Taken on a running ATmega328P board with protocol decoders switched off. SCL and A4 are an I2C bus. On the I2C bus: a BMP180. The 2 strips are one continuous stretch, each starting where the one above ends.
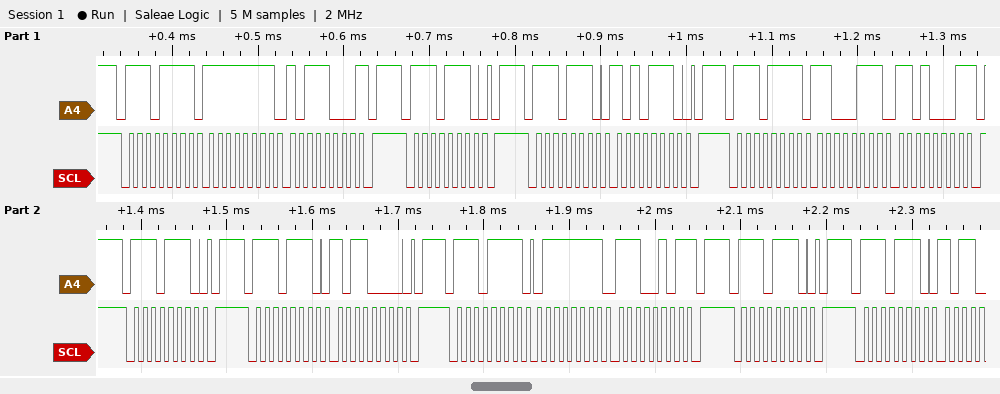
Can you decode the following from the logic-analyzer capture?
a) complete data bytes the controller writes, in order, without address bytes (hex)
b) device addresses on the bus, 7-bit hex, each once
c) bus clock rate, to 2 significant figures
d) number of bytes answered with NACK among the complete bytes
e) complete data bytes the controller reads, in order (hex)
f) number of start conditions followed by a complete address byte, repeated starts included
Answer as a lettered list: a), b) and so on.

a) AE B0
b) 0x77
c) 100 kHz
d) 3
e) FF B8 C7 D1 7F E5
f) 9
